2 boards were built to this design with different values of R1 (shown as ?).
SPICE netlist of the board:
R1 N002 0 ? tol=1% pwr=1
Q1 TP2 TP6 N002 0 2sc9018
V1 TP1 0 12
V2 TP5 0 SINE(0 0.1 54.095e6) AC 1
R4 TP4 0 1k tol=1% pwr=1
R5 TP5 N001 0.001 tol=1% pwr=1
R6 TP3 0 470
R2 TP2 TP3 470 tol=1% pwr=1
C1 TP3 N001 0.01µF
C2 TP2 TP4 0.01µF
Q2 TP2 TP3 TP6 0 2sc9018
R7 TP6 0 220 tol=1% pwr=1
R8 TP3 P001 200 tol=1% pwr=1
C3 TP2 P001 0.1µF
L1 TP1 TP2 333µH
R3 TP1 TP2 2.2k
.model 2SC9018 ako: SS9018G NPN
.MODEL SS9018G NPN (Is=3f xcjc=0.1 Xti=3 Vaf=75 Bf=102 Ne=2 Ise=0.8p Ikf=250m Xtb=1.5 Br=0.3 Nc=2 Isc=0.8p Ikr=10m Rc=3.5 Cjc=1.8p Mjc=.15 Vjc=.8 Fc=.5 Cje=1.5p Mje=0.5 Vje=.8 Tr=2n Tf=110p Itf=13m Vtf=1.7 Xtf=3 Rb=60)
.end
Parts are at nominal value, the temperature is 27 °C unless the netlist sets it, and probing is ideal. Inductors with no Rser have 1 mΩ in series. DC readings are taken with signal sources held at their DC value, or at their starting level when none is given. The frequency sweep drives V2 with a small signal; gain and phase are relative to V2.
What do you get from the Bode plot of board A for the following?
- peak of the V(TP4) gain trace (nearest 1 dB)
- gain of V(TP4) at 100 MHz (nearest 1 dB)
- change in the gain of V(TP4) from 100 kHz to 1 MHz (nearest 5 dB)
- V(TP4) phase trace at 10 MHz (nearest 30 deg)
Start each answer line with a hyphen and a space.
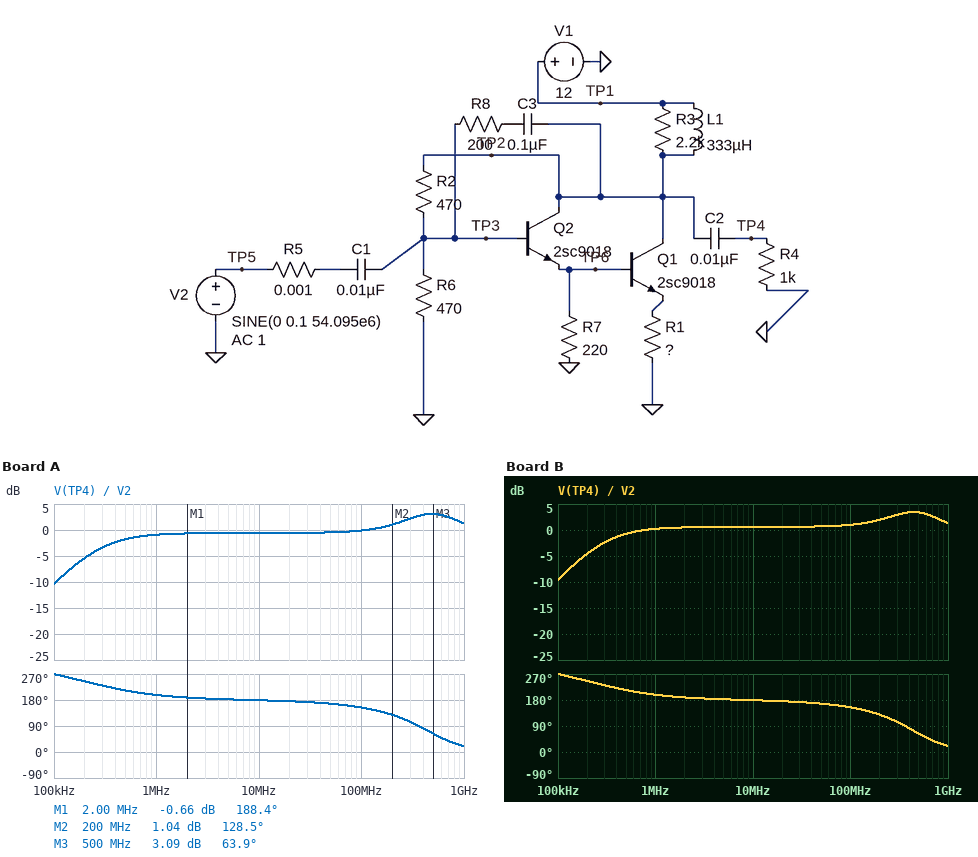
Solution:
- 3 dB
- 0 dB
- 10 dB
- 180 deg
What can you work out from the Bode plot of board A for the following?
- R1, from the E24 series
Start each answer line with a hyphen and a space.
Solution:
- 91 Ω
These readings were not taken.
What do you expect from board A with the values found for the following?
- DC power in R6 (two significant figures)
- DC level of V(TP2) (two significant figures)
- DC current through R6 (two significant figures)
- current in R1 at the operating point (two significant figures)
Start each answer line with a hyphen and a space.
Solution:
- 75 mW
- 12 V
- 13 mA
- 48 mA
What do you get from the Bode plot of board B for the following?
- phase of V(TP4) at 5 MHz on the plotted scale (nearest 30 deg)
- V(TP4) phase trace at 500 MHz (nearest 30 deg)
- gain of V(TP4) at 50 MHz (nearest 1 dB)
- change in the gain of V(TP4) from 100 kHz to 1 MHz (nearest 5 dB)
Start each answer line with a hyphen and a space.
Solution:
- 180 deg
- 60 deg
- 1 dB
- 10 dB
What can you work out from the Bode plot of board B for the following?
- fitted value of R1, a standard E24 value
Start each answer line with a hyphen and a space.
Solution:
- 82 Ω
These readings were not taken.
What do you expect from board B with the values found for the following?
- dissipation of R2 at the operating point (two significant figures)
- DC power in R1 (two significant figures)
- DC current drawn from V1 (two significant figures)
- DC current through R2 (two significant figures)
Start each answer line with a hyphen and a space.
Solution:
- 78 mW
- 230 mW
- 89 mA
- 13 mA
